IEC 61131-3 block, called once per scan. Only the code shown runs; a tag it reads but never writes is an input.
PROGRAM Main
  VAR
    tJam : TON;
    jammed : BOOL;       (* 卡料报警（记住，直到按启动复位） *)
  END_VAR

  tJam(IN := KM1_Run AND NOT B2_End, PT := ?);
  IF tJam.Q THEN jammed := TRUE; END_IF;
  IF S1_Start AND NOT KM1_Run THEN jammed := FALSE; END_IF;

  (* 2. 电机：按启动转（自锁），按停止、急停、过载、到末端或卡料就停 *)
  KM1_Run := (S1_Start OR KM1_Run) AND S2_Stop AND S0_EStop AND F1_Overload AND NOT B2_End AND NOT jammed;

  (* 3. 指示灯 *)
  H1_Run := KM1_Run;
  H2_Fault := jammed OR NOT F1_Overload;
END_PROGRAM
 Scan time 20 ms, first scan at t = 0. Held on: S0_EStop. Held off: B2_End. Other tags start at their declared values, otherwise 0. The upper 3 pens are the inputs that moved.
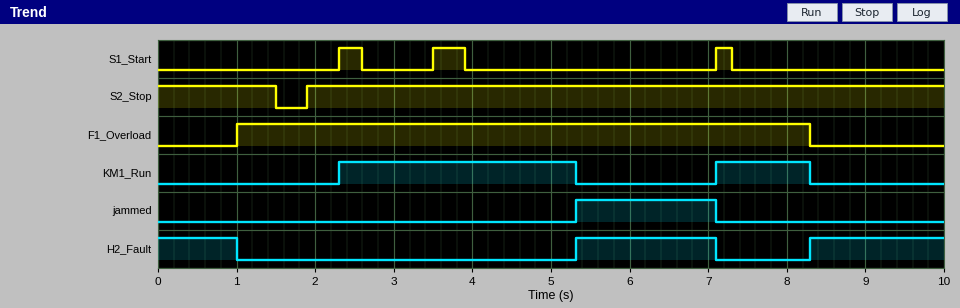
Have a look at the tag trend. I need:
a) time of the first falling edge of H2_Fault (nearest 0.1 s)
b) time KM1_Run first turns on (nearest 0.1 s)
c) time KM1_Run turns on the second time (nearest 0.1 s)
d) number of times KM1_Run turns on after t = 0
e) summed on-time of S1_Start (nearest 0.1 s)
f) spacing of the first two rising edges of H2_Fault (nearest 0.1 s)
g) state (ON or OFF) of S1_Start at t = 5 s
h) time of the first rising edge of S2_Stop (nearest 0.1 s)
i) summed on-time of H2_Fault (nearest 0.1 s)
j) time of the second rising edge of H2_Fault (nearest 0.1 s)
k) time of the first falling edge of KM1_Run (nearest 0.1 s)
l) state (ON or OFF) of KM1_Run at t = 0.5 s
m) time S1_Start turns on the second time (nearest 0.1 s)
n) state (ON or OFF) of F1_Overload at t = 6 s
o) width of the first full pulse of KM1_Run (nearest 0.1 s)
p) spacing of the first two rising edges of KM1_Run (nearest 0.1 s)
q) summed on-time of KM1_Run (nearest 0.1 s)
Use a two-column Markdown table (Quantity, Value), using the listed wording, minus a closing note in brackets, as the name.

| Quantity | Value |
|---|---|
| time of the first falling edge of H2_Fault | 1.0 s |
| time KM1_Run first turns on | 2.3 s |
| time KM1_Run turns on the second time | 7.1 s |
| number of times KM1_Run turns on after t = 0 | 2 |
| summed on-time of S1_Start | 0.9 s |
| spacing of the first two rising edges of H2_Fault | 3.0 s |
| state (ON or OFF) of S1_Start at t = 5 s | OFF |
| time of the first rising edge of S2_Stop | 1.9 s |
| summed on-time of H2_Fault | 4.5 s |
| time of the second rising edge of H2_Fault | 8.3 s |
| time of the first falling edge of KM1_Run | 5.3 s |
| state (ON or OFF) of KM1_Run at t = 0.5 s | OFF |
| time S1_Start turns on the second time | 3.5 s |
| state (ON or OFF) of F1_Overload at t = 6 s | ON |
| width of the first full pulse of KM1_Run | 3.0 s |
| spacing of the first two rising edges of KM1_Run | 4.8 s |
| summed on-time of KM1_Run | 4.2 s |
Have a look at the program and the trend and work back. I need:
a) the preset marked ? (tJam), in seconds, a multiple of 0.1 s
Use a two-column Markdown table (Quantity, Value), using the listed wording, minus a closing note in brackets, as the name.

| Quantity | Value |
|---|---|
| the preset marked ? (tJam), in seconds, a multiple of 0.1 s | 3.0 s |
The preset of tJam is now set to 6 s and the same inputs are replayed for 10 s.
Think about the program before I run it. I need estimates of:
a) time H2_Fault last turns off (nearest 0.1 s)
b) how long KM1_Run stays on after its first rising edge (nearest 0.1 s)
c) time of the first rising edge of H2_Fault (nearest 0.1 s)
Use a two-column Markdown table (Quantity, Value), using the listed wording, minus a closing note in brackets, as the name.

| Quantity | Value |
|---|---|
| time H2_Fault last turns off | 1.0 s |
| how long KM1_Run stays on after its first rising edge | 6.0 s |
| time of the first rising edge of H2_Fault | 8.3 s |
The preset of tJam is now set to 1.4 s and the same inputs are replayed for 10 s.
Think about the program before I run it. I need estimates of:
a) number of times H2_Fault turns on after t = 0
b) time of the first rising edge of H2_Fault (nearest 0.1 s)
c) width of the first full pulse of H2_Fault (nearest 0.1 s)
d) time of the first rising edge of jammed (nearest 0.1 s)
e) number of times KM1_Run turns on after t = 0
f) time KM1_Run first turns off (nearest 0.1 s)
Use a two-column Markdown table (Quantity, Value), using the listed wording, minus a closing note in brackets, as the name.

| Quantity | Value |
|---|---|
| number of times H2_Fault turns on after t = 0 | 3 |
| time of the first rising edge of H2_Fault | 3.7 s |
| width of the first full pulse of H2_Fault | 0.0 s |
| time of the first rising edge of jammed | 3.7 s |
| number of times KM1_Run turns on after t = 0 | 3 |
| time KM1_Run first turns off | 3.7 s |
